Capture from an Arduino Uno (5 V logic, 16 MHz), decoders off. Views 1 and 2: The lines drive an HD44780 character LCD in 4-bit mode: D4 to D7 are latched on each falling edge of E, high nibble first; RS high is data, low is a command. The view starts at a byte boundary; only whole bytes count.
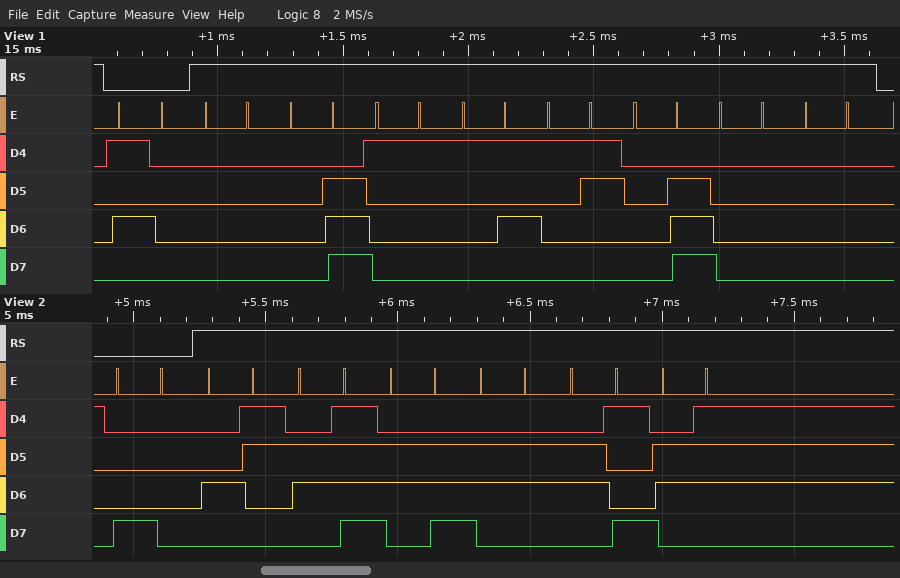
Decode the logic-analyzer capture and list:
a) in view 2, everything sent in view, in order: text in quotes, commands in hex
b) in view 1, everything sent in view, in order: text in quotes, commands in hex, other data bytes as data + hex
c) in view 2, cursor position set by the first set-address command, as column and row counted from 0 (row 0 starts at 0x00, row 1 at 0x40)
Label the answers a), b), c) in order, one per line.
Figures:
a) 0x80 "Config"
b) 0x50 data 00 0E 11 15 13 0E 00 00
c) column 0, row 0
